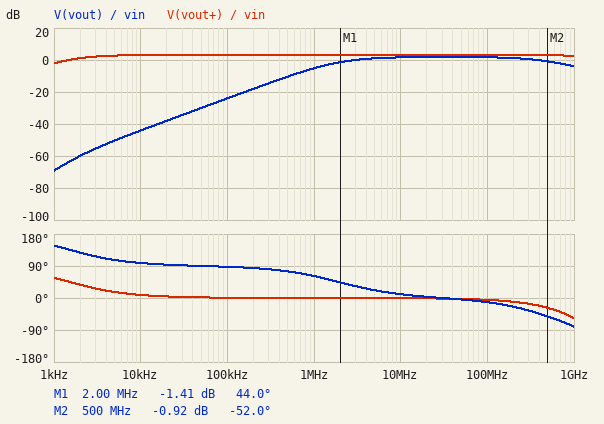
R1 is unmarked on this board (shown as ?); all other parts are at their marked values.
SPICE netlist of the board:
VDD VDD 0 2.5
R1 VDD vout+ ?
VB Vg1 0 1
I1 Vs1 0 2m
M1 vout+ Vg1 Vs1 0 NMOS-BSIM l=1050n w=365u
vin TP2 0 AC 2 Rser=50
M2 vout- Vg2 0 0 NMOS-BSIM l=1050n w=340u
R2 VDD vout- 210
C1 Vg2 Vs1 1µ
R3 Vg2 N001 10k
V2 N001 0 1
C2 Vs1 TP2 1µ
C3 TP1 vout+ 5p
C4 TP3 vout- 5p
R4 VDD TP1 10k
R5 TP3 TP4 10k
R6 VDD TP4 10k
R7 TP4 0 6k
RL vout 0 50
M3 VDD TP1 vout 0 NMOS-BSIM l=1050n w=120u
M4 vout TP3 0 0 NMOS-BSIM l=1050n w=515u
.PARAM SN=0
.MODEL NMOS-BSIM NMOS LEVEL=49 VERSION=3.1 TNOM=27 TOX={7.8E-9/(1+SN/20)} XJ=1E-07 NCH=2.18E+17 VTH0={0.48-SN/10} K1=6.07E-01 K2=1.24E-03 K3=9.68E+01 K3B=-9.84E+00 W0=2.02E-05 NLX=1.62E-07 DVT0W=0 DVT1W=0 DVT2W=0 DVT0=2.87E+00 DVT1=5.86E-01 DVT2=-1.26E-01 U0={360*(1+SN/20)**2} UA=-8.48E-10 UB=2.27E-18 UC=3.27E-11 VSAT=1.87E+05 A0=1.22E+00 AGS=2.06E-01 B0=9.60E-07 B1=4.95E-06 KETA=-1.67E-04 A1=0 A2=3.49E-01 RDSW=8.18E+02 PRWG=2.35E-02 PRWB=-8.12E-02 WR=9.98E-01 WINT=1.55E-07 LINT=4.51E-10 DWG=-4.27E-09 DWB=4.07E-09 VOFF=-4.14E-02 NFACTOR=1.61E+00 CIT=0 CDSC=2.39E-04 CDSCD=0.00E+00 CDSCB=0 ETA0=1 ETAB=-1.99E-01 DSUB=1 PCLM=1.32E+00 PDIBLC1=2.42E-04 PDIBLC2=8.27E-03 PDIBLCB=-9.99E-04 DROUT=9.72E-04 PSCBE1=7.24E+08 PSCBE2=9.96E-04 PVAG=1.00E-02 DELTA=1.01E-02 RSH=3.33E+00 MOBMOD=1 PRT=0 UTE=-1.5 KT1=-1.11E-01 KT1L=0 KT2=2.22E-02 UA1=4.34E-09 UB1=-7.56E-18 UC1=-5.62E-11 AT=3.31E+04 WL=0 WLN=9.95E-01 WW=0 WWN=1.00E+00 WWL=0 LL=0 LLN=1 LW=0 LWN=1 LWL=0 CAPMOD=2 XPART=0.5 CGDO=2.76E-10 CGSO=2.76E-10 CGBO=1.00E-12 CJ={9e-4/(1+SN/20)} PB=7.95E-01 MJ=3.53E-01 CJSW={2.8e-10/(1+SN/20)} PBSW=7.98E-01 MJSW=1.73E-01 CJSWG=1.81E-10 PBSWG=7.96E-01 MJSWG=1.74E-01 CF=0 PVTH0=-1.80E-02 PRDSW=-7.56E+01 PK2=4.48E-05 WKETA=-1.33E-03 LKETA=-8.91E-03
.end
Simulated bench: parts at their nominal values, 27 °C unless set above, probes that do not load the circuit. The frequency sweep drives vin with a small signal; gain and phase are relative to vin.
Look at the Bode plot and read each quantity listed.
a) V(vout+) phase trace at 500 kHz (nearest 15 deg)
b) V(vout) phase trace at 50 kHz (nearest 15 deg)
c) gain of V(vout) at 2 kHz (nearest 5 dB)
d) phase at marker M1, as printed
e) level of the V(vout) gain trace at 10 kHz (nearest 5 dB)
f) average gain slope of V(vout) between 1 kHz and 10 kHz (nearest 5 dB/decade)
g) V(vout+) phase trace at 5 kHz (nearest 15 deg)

0 deg
90 deg
-60 dB
44.0 deg
-45 dB
25 dB/decade
15 deg
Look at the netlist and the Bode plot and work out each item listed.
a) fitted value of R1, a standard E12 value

150 Ω
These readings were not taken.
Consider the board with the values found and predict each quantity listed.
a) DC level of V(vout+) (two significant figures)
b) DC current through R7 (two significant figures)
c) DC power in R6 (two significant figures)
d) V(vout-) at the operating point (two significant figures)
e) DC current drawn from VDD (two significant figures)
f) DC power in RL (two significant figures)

2.2 V
160 µA
240 µW
1.5 V
20 mA
3.1 mW
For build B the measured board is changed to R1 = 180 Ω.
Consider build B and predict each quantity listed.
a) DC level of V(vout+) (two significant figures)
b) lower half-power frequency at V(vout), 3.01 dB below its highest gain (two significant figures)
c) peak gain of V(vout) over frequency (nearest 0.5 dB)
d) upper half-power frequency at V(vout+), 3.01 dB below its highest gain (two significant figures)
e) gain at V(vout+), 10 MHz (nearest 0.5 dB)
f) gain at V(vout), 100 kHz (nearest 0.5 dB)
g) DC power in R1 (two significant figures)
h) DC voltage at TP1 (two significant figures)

2.1 V
2.2 MHz
2.5 dB
1.7 GHz
4.5 dB
-23.5 dB
720 µW
2.5 V
